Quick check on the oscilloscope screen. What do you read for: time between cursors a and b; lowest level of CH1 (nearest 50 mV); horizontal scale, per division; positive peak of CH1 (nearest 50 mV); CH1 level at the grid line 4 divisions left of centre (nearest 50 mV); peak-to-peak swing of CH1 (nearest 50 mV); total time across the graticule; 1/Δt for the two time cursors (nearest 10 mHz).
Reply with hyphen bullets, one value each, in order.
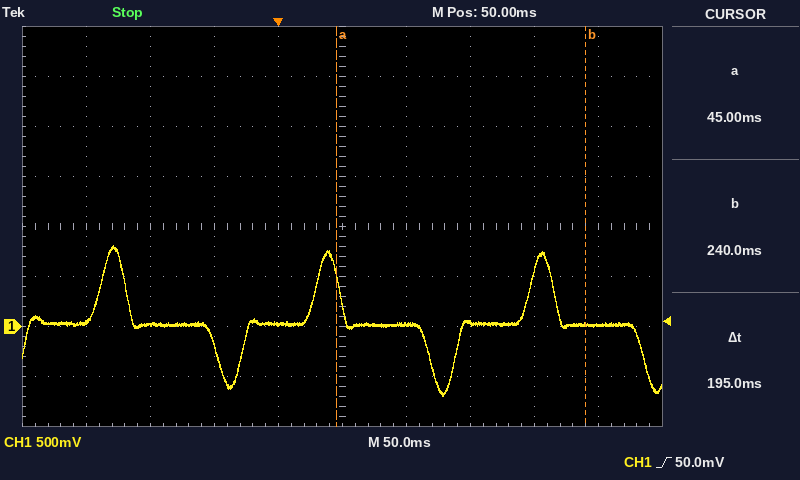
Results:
- 195 ms
- -700 mV
- 50 ms
- 800 mV
- 50 mV
- 1.50 V
- 500 ms
- 5.13 Hz
